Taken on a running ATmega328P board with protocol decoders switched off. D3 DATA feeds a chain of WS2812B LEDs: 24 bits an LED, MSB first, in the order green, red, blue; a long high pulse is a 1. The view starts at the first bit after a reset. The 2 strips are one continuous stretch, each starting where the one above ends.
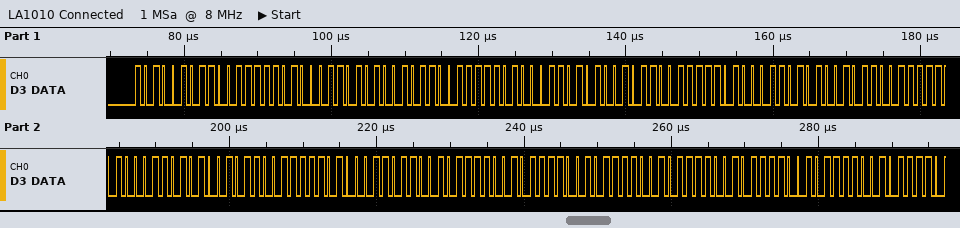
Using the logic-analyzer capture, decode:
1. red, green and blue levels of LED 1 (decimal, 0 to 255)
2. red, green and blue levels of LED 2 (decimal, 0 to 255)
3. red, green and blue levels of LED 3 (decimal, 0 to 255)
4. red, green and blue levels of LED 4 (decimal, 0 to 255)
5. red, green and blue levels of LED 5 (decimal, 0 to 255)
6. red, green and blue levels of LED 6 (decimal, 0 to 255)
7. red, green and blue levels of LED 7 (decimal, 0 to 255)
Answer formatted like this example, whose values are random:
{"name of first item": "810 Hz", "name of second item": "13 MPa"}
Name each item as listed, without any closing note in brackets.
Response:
{"red, green and blue levels of LED 1": "159, 165, 70", "red, green and blue levels of LED 2": "159, 165, 70", "red, green and blue levels of LED 3": "159, 165, 70", "red, green and blue levels of LED 4": "159, 165, 70", "red, green and blue levels of LED 5": "159, 165, 70", "red, green and blue levels of LED 6": "203, 203, 203", "red, green and blue levels of LED 7": "203, 203, 203"}
